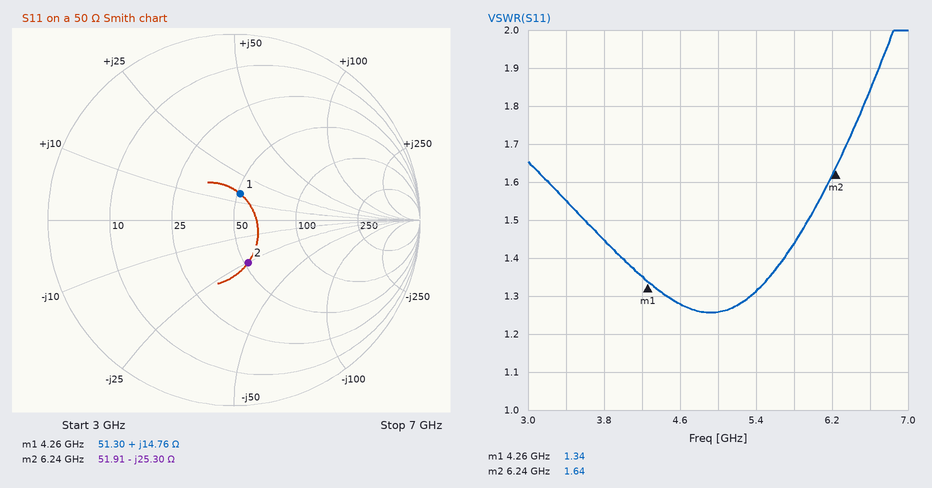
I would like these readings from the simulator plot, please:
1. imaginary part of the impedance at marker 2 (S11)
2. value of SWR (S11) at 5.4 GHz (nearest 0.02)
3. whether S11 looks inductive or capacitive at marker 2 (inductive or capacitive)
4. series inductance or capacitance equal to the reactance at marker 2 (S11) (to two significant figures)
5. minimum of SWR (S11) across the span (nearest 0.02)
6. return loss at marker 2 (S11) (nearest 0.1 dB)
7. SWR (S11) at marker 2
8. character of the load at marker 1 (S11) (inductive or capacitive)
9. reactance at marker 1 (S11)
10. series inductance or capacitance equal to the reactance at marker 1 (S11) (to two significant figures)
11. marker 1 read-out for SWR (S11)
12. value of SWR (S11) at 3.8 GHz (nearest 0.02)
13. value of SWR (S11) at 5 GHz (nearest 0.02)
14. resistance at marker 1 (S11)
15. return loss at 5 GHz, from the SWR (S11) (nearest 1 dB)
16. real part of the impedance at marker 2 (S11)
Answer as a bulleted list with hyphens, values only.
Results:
- -25.30 Ω
- 1.32
- capacitive
- 1.0 pF
- 1.26
- 12.3 dB
- 1.64
- inductive
- +14.76 Ω
- 550 pH
- 1.34
- 1.44
- 1.26
- 51.30 Ω
- 19 dB
- 51.91 Ω
